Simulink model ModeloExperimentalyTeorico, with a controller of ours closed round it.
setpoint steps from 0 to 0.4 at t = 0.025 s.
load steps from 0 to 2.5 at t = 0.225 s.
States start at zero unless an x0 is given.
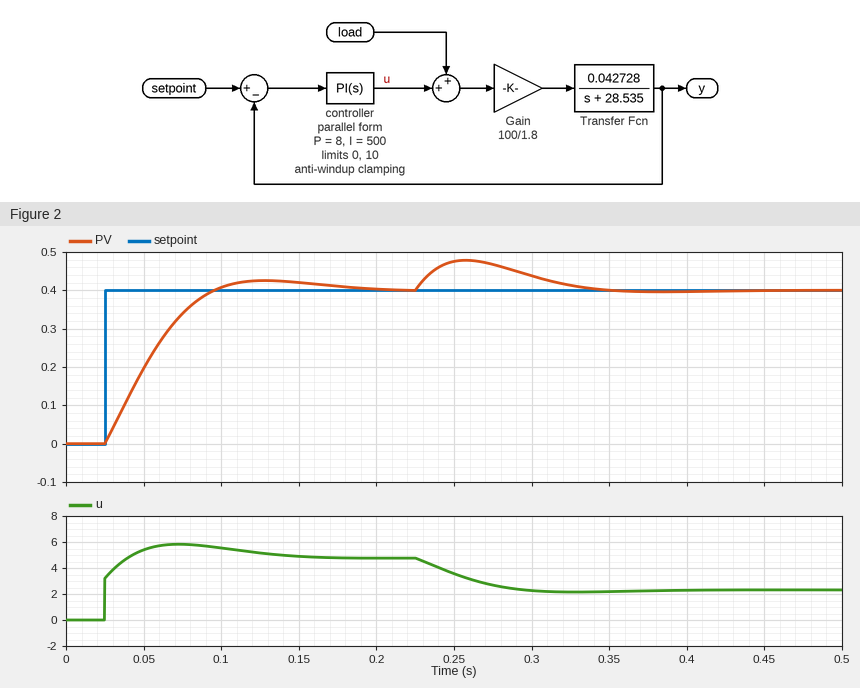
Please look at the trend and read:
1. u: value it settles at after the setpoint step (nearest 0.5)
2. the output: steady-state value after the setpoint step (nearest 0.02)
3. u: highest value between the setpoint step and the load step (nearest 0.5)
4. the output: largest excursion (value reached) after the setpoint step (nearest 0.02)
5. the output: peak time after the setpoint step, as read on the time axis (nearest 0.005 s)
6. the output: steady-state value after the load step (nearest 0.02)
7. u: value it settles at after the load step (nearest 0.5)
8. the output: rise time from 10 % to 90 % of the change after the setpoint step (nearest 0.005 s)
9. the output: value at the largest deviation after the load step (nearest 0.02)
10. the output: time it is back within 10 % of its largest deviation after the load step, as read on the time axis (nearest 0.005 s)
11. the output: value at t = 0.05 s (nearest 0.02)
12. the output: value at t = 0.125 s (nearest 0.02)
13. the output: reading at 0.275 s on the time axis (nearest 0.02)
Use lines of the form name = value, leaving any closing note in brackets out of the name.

u: value it settles at after the setpoint step = 5.0
the output: steady-state value after the setpoint step = 0.40
u: highest value between the setpoint step and the load step = 6.0
the output: largest excursion (value reached) after the setpoint step = 0.42
the output: peak time after the setpoint step, as read on the time axis = 0.130 s
the output: steady-state value after the load step = 0.40
u: value it settles at after the load step = 2.5
the output: rise time from 10 % to 90 % of the change after the setpoint step = 0.050 s
the output: value at the largest deviation after the load step = 0.48
the output: time it is back within 10 % of its largest deviation after the load step, as read on the time axis = 0.335 s
the output: value at t = 0.05 s = 0.20
the output: value at t = 0.125 s = 0.42
the output: reading at 0.275 s on the time axis = 0.46
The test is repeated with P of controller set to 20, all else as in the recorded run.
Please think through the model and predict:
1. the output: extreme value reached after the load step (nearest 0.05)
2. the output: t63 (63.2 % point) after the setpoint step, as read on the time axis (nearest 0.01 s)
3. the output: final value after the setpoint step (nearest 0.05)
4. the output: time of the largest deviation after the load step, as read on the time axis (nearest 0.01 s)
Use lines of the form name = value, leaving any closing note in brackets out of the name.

the output: extreme value reached after the load step = 0.45
the output: t63 (63.2 % point) after the setpoint step, as read on the time axis = 0.05 s
the output: final value after the setpoint step = 0.40
the output: time of the largest deviation after the load step, as read on the time axis = 0.25 s
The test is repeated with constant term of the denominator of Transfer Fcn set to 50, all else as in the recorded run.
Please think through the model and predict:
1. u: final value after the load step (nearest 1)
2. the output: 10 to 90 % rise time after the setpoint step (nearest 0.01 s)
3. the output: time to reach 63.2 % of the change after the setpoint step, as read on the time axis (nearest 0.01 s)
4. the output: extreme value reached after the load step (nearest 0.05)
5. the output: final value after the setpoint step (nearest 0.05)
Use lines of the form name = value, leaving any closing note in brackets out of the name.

u: final value after the load step = 6
the output: 10 to 90 % rise time after the setpoint step = 0.09 s
the output: time to reach 63.2 % of the change after the setpoint step, as read on the time axis = 0.07 s
the output: extreme value reached after the load step = 0.45
the output: final value after the setpoint step = 0.40
